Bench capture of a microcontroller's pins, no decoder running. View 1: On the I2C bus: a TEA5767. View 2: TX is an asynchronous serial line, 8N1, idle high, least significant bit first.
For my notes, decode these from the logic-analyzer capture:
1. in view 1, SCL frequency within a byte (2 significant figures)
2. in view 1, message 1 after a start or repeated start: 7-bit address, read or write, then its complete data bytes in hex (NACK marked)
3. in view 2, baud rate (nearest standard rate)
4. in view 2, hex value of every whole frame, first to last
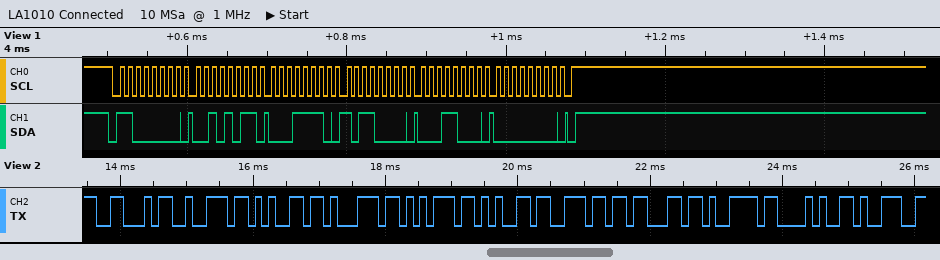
100 kHz
0x60 write: 2B 1E B0 18 00
9600 baud
0x46 0x72 0x65 0x71 0x75 0x65 0x6E 0x63 0x79 0x28 0x39
